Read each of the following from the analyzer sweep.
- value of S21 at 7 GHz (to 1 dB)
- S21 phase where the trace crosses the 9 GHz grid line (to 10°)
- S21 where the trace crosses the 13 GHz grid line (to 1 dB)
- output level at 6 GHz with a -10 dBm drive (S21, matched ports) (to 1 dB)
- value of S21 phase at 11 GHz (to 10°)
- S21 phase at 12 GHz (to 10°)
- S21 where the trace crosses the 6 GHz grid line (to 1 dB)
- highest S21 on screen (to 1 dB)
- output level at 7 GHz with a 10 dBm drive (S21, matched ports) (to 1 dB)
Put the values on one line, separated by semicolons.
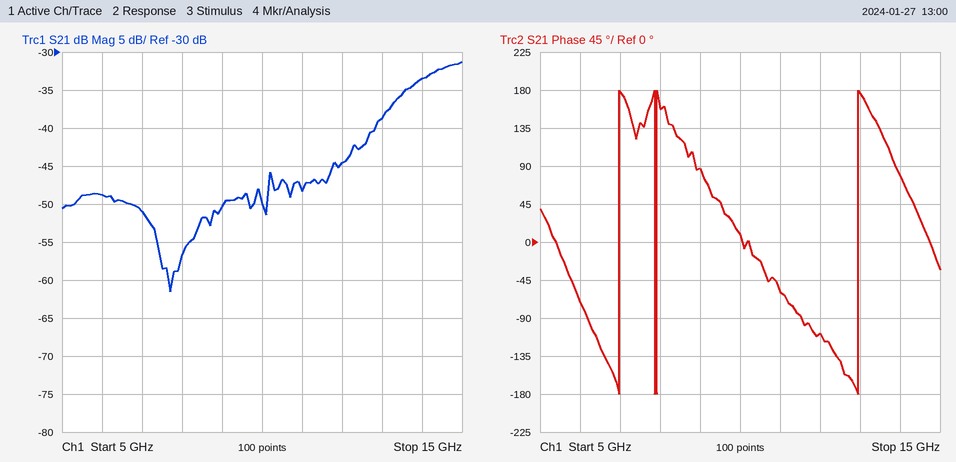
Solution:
-51 dB; 90°; -39 dB; -59 dBm; -60°; -110°; -49 dB; -31 dB; -41 dBm
